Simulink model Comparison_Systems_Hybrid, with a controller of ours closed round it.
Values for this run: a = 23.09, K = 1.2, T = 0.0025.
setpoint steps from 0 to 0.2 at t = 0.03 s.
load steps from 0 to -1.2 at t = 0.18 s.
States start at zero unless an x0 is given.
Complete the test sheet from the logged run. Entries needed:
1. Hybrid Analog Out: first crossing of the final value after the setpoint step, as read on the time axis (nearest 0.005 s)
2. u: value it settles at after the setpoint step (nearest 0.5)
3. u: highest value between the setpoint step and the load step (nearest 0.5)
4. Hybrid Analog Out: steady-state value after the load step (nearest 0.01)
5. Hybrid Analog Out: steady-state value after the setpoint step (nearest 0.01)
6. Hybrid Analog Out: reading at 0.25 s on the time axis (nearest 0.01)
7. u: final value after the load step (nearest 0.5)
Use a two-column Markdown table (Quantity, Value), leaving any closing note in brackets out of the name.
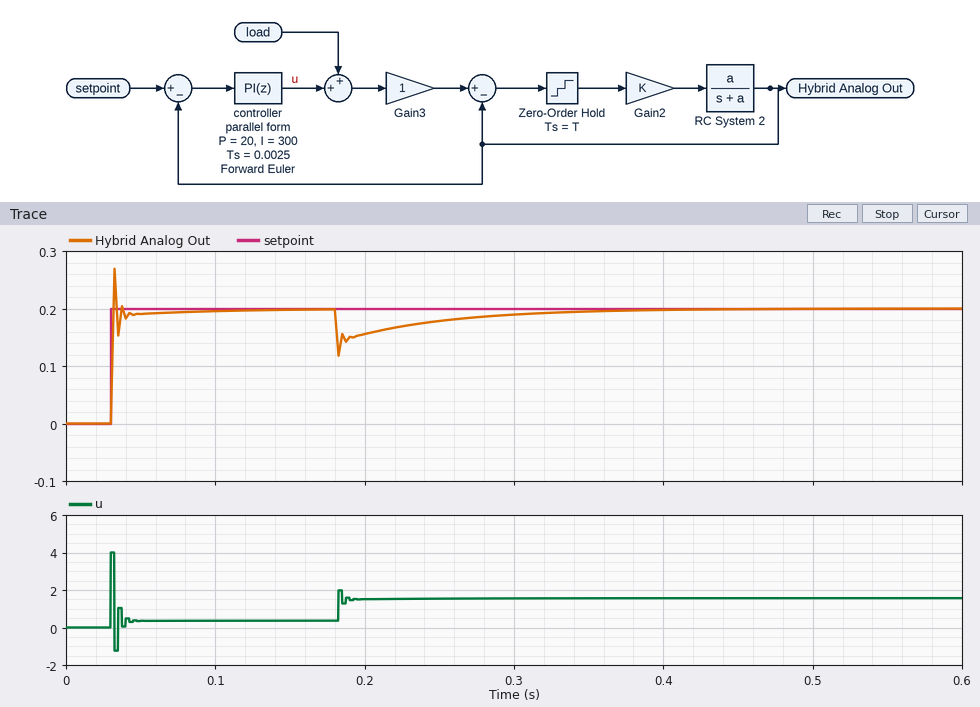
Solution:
| Quantity | Value |
|---|---|
| Hybrid Analog Out: first crossing of the final value after the setpoint step, as read on the time axis | 0.030 s |
| u: value it settles at after the setpoint step | 0.5 |
| u: highest value between the setpoint step and the load step | 4.0 |
| Hybrid Analog Out: steady-state value after the load step | 0.20 |
| Hybrid Analog Out: steady-state value after the setpoint step | 0.20 |
| Hybrid Analog Out: reading at 0.25 s on the time axis | 0.18 |
| u: final value after the load step | 1.5 |
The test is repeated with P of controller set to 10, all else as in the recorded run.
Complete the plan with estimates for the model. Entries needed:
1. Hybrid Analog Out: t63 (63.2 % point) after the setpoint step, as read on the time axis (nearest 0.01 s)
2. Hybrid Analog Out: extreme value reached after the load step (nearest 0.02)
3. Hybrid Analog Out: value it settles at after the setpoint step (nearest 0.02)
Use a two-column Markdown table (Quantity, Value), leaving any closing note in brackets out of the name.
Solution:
| Quantity | Value |
|---|---|
| Hybrid Analog Out: t63 (63.2 % point) after the setpoint step, as read on the time axis | 0.03 s |
| Hybrid Analog Out: extreme value reached after the load step | 0.10 |
| Hybrid Analog Out: value it settles at after the setpoint step | 0.20 |
